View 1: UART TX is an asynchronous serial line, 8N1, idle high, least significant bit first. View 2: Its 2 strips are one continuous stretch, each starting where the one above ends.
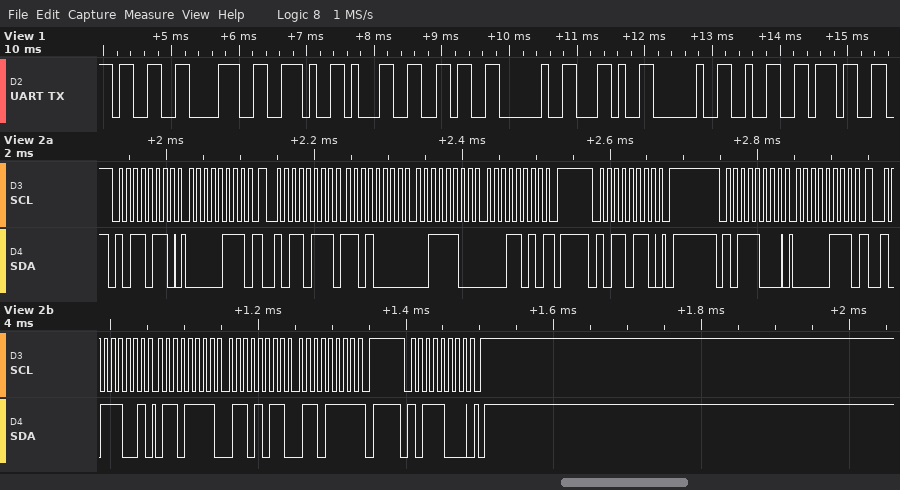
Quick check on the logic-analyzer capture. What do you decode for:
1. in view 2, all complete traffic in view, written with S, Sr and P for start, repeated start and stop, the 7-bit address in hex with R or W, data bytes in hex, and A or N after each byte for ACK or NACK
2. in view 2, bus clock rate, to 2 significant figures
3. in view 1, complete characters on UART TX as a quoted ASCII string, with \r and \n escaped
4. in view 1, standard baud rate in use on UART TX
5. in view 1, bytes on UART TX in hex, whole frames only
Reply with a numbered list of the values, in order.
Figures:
1. S 5BW A 07 A Sr 5BR A D0 A 3C A 1A N P S 5BW A P S 5CW A 07 A Sr 5CR A 6F A 6B A 6F N P S 5CW A P
2. 100 kHz
3. "38.16 , 27"
4. 9600 baud
5. 33 38 2E 31 36 20 2C 20 32 37
